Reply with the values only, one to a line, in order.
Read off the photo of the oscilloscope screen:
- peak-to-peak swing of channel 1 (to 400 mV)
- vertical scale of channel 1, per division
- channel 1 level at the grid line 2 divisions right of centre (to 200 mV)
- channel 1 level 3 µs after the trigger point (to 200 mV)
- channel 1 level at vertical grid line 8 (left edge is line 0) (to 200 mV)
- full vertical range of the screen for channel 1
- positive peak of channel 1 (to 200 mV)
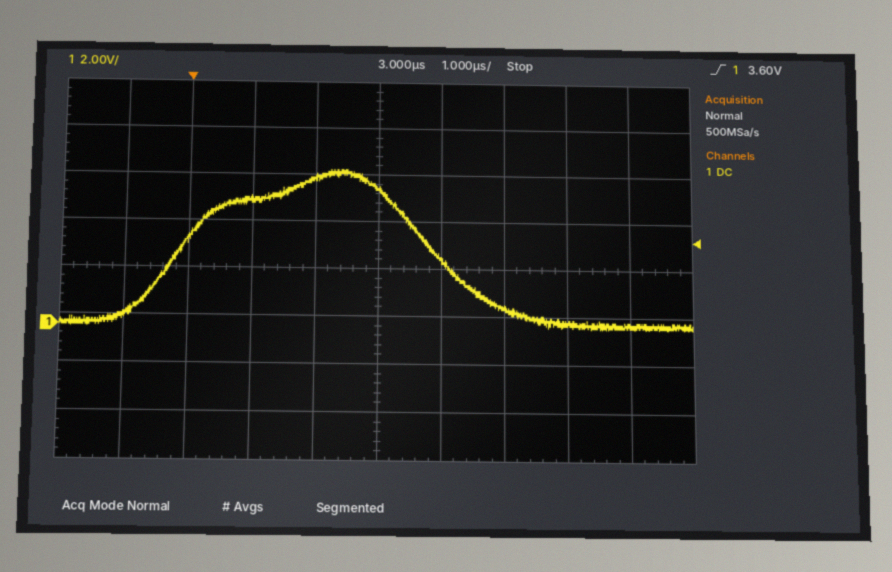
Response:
6.8 V
2 V
800 mV
5.8 V
200 mV
16 V
6.6 V
